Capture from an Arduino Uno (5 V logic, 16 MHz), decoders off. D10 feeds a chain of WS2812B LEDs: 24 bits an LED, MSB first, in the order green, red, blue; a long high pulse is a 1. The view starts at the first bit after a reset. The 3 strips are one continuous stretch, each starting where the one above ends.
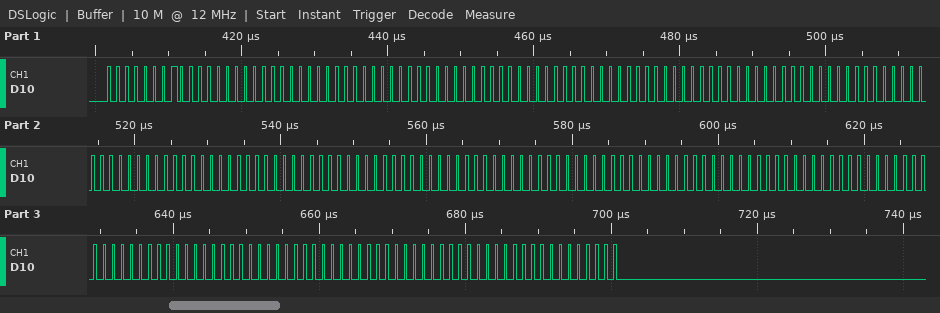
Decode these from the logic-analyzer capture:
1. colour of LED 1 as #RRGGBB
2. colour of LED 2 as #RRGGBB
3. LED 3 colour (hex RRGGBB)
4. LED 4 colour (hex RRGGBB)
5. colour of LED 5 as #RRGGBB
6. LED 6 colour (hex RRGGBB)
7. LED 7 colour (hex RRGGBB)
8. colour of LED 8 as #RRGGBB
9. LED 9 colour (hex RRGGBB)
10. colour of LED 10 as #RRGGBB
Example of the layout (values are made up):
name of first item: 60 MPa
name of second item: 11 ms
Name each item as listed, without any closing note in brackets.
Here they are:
colour of LED 1 as #RRGGBB: #000100
colour of LED 2 as #RRGGBB: #000000
LED 3 colour: #000000
LED 4 colour: #000000
colour of LED 5 as #RRGGBB: #000000
LED 6 colour: #000000
LED 7 colour: #000000
colour of LED 8 as #RRGGBB: #000000
LED 9 colour: #000000
colour of LED 10 as #RRGGBB: #000000
